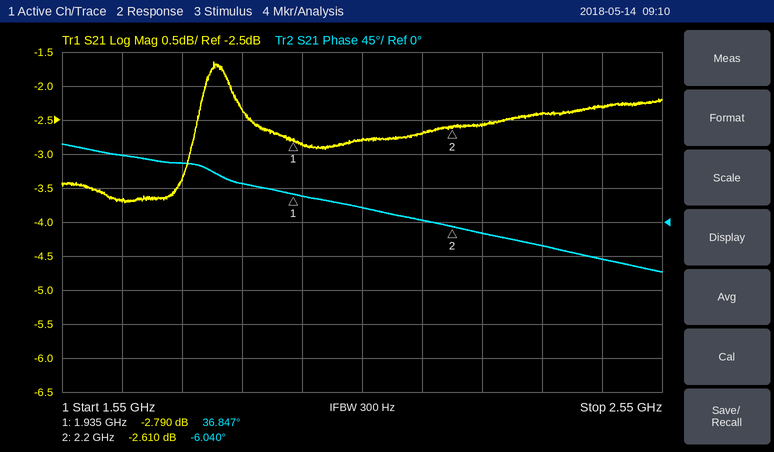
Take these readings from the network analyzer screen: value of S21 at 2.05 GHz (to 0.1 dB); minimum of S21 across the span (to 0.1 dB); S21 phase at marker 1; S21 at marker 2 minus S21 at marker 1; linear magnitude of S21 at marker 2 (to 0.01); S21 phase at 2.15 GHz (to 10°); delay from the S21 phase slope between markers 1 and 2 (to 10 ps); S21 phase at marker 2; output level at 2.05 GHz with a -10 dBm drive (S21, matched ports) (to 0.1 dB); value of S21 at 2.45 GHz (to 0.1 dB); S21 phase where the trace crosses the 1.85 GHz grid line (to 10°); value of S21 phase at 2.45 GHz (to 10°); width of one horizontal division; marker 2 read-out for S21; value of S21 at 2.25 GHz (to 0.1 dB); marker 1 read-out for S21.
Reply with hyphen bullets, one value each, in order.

- -2.8 dB
- -3.7 dB
- 36.847°
- 0.180 dB
- 0.74
- 0°
- 450 ps
- -6.040°
- -12.8 dBm
- -2.3 dB
- 50°
- -50°
- 100 MHz
- -2.610 dB
- -2.6 dB
- -2.790 dB
